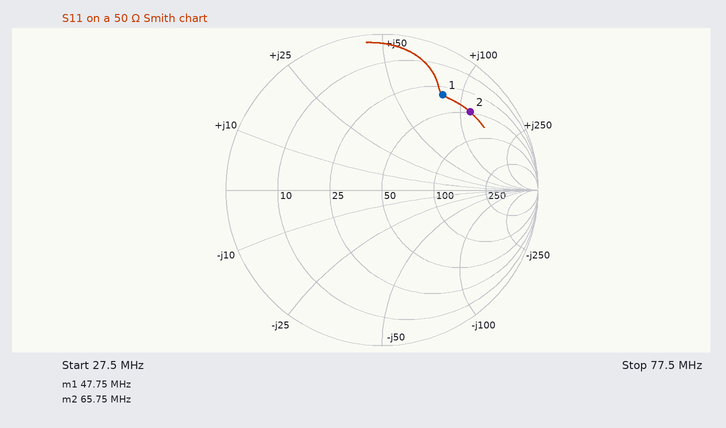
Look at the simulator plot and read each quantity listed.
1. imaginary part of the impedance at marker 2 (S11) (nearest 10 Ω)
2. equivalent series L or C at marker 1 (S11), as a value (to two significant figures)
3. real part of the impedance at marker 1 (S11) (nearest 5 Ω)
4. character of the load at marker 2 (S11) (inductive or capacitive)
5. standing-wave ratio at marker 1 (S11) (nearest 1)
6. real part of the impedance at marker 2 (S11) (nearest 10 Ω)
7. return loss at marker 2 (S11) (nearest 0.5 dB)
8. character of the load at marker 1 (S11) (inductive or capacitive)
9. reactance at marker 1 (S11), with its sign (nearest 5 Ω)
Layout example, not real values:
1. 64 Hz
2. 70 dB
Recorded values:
1. +110 Ω
2. 270 nH
3. 30 Ω
4. inductive
5. 6
6. 50 Ω
7. 2.5 dB
8. inductive
9. +80 Ω
